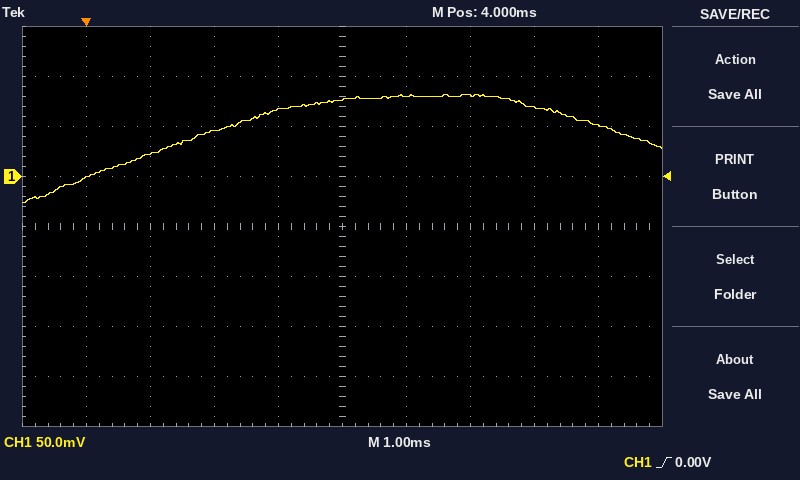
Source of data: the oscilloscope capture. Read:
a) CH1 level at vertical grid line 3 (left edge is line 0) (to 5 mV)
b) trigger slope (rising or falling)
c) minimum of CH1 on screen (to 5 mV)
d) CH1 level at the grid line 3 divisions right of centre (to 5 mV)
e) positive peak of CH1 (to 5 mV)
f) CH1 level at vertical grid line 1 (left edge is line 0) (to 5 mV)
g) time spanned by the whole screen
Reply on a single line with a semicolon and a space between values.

45 mV; rising; -25 mV; 70 mV; 80 mV; 0 mV; 10 ms
